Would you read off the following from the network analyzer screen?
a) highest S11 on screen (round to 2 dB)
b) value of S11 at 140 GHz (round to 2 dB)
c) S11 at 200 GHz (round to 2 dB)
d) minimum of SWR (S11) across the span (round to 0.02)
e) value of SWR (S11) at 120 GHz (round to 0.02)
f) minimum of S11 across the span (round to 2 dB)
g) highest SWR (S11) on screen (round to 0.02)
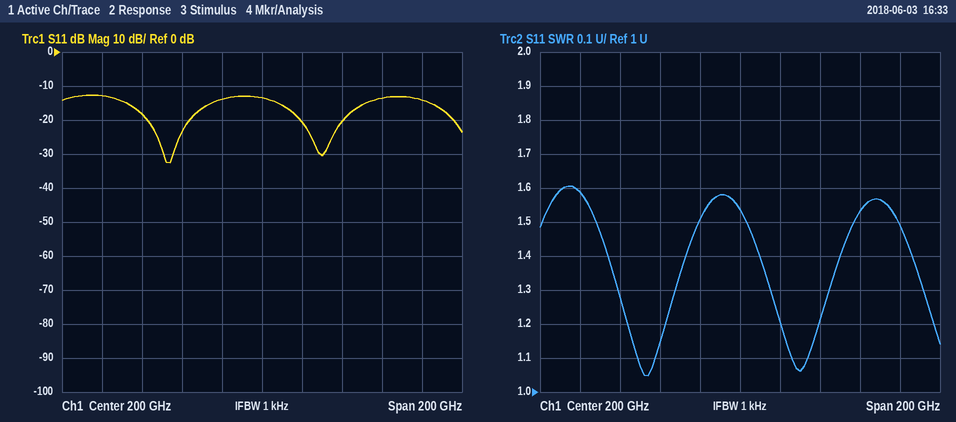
-12 dB
-18 dB
-14 dB
1.04
1.58
-32 dB
1.60
